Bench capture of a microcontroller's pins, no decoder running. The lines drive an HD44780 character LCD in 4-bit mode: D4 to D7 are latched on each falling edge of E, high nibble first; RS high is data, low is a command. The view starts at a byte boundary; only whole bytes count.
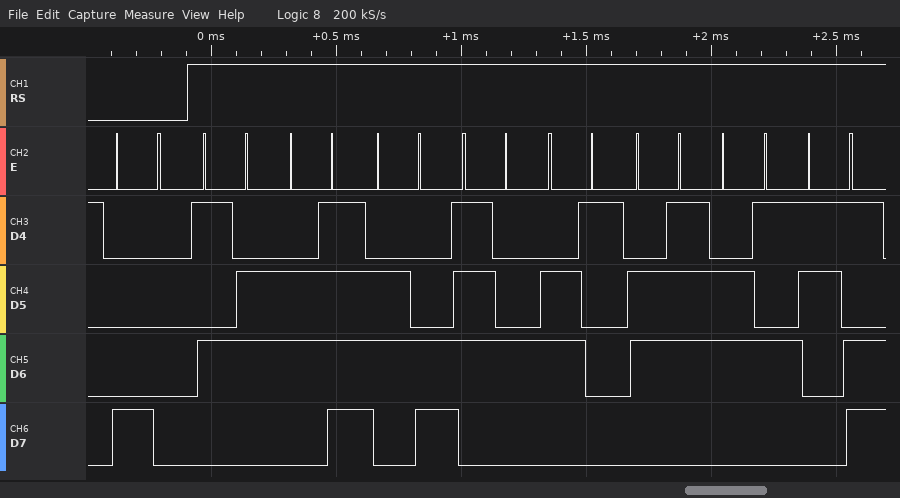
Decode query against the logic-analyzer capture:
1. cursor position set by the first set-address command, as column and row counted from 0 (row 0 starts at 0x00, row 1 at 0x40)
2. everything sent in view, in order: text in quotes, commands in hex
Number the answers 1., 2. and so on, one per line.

1. column 0, row 0
2. 0x80 "Voltage="
